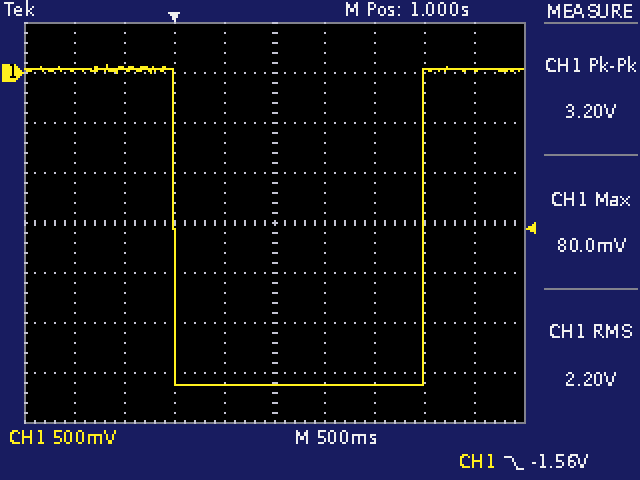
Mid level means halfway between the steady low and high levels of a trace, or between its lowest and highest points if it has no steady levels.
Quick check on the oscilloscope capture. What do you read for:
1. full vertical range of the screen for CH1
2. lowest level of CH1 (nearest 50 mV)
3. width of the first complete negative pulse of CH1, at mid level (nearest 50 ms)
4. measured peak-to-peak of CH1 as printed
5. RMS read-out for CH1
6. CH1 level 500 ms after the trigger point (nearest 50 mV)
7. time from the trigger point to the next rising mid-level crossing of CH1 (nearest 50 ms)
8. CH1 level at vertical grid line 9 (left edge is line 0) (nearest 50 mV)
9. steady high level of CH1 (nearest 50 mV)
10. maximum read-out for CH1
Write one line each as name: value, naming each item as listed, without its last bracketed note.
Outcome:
full vertical range of the screen for CH1: 4 V
lowest level of CH1: -3.10 V
width of the first complete negative pulse of CH1, at mid level: 2.50 s
measured peak-to-peak of CH1 as printed: 3.20 V
RMS read-out for CH1: 2.20 V
CH1 level 500 ms after the trigger point: -3.10 V
time from the trigger point to the next rising mid-level crossing of CH1: 2.50 s
CH1 level at vertical grid line 9 (left edge is line 0): 50 mV
steady high level of CH1: 50 mV
maximum read-out for CH1: 80.0 mV
